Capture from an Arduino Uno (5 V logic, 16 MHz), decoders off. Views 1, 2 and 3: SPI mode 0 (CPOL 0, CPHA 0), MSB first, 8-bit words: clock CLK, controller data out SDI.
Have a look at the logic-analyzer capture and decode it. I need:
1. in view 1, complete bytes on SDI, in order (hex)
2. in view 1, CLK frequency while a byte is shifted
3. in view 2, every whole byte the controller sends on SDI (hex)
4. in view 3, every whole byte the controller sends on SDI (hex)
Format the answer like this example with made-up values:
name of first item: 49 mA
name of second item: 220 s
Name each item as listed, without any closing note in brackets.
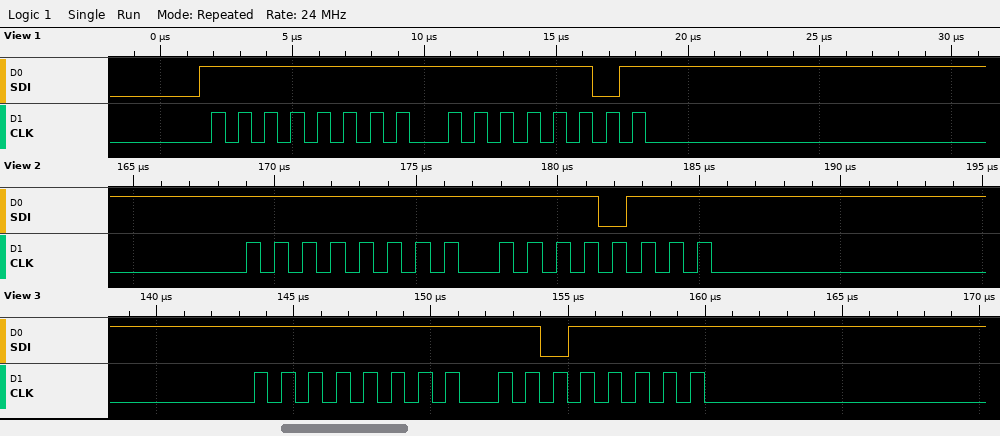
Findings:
in view 1, complete bytes on SDI, in order: FF FD
in view 1, CLK frequency while a byte is shifted: 1 MHz
in view 2, every whole byte the controller sends on SDI: FF F7
in view 3, every whole byte the controller sends on SDI: 0xFF 0xDF
